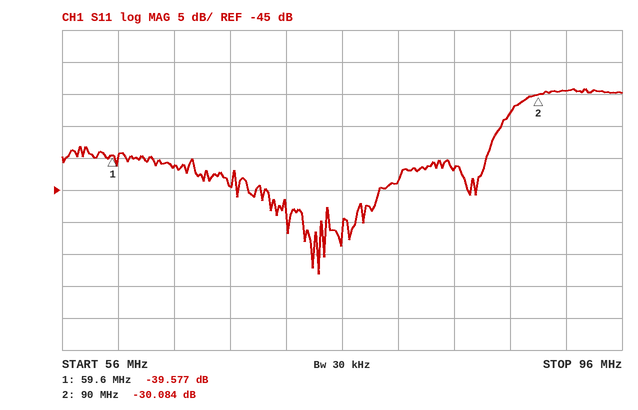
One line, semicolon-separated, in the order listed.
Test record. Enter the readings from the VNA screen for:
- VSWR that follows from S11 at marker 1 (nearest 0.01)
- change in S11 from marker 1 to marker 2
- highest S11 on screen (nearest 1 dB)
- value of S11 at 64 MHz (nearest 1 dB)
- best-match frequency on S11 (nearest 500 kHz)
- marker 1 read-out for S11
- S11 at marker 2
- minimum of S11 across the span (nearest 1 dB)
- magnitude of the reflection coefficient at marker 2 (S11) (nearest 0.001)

1.02; 9.493 dB; -29 dB; -41 dB; 74.5 MHz; -39.577 dB; -30.084 dB; -58 dB; 0.031
